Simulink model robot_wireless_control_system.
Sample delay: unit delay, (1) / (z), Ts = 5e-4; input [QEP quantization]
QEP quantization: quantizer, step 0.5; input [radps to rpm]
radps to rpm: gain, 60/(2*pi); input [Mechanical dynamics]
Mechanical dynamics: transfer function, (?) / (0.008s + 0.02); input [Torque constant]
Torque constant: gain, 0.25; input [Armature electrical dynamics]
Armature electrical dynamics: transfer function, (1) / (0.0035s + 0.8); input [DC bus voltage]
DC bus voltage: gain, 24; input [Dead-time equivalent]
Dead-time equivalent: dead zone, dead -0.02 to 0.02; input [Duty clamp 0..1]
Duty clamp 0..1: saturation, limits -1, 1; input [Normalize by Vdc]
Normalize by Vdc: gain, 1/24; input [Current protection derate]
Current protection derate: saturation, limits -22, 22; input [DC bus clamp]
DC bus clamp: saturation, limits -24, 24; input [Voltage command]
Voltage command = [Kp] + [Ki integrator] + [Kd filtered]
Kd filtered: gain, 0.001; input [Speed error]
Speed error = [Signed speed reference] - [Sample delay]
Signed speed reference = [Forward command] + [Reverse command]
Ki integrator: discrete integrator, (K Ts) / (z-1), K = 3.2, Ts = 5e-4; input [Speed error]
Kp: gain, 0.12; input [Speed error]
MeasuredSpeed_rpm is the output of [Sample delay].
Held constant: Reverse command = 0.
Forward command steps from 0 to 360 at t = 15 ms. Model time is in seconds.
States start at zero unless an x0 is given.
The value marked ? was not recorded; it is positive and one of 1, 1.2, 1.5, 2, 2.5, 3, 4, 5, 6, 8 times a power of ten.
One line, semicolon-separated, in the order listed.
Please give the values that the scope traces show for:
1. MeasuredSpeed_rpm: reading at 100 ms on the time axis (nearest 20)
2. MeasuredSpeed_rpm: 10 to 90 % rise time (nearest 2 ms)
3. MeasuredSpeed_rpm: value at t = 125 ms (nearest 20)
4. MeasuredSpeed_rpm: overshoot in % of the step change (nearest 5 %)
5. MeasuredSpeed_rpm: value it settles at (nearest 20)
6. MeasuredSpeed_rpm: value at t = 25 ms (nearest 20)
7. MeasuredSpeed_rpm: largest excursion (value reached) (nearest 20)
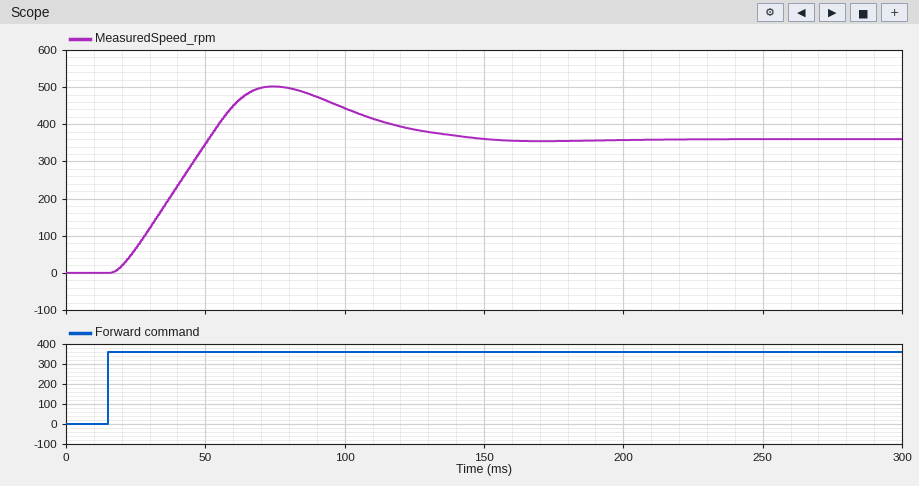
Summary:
440; 26 ms; 380; 40 %; 360; 60; 500
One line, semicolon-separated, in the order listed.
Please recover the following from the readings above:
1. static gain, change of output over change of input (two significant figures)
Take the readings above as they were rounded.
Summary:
1.0
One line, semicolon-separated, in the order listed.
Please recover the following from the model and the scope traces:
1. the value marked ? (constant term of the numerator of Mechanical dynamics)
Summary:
1.5
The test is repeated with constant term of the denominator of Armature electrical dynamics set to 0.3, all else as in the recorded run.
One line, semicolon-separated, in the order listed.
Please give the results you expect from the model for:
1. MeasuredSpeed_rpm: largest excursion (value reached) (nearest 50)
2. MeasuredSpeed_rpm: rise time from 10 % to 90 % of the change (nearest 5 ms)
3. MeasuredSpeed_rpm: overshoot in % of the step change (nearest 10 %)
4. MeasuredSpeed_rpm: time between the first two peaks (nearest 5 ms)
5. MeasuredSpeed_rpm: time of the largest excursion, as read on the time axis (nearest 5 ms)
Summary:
600; 15 ms; 60 %; 55 ms; 50 ms
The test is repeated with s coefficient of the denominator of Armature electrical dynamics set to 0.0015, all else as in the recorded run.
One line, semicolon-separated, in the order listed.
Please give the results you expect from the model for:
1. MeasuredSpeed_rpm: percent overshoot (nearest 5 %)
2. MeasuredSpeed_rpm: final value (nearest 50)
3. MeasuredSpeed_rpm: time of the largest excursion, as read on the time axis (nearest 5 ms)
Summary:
30 %; 350; 70 ms
